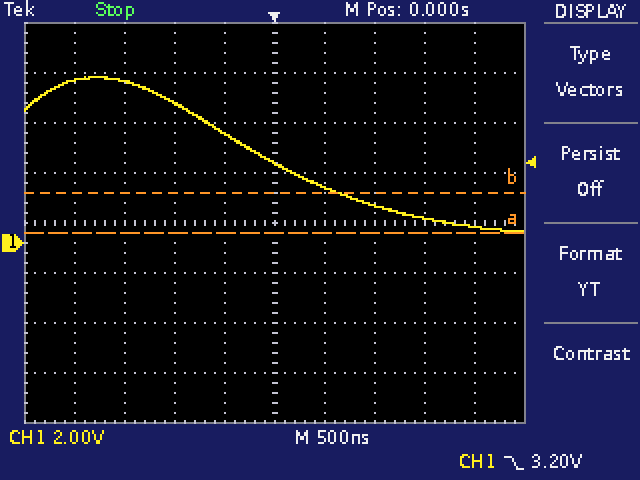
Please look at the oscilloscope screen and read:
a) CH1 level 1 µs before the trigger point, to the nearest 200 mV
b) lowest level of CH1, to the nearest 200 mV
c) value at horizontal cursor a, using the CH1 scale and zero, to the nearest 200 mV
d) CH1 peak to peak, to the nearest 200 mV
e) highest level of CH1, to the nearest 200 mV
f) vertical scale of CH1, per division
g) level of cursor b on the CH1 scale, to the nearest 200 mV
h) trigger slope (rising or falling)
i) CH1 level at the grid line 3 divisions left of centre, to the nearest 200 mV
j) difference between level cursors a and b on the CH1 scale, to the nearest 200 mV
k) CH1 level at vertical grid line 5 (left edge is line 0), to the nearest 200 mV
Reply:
5.6 V
400 mV
400 mV
6.2 V
6.6 V
2 V
2.0 V
falling
6.4 V
1.6 V
3.2 V
